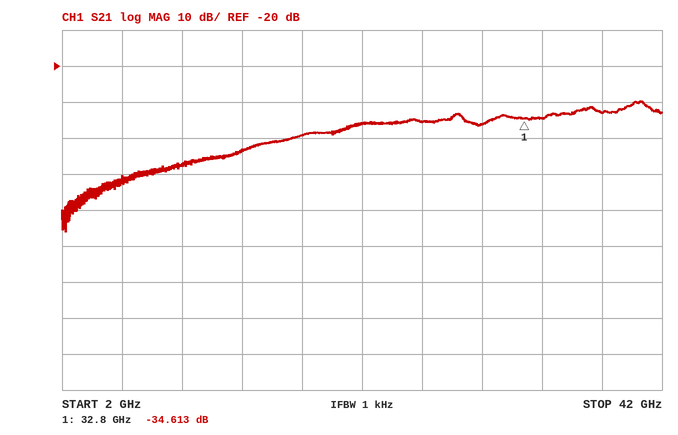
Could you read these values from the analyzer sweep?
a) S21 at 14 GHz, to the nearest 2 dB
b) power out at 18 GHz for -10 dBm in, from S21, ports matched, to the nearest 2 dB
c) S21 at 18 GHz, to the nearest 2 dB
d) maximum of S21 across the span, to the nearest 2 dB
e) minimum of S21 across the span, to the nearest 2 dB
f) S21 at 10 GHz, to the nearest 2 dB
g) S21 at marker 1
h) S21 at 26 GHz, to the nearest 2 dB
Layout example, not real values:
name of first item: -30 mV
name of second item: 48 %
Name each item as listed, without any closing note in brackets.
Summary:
S21 at 14 GHz, to the nearest 2 dB: -44 dB
power out at 18 GHz for -10 dBm in, from S21, ports matched, to the nearest 2 dB: -50 dBm
S21 at 18 GHz, to the nearest 2 dB: -40 dB
maximum of S21 across the span, to the nearest 2 dB: -30 dB
minimum of S21 across the span, to the nearest 2 dB: -66 dB
S21 at 10 GHz, to the nearest 2 dB: -48 dB
S21 at marker 1: -34.613 dB
S21 at 26 GHz, to the nearest 2 dB: -36 dB
